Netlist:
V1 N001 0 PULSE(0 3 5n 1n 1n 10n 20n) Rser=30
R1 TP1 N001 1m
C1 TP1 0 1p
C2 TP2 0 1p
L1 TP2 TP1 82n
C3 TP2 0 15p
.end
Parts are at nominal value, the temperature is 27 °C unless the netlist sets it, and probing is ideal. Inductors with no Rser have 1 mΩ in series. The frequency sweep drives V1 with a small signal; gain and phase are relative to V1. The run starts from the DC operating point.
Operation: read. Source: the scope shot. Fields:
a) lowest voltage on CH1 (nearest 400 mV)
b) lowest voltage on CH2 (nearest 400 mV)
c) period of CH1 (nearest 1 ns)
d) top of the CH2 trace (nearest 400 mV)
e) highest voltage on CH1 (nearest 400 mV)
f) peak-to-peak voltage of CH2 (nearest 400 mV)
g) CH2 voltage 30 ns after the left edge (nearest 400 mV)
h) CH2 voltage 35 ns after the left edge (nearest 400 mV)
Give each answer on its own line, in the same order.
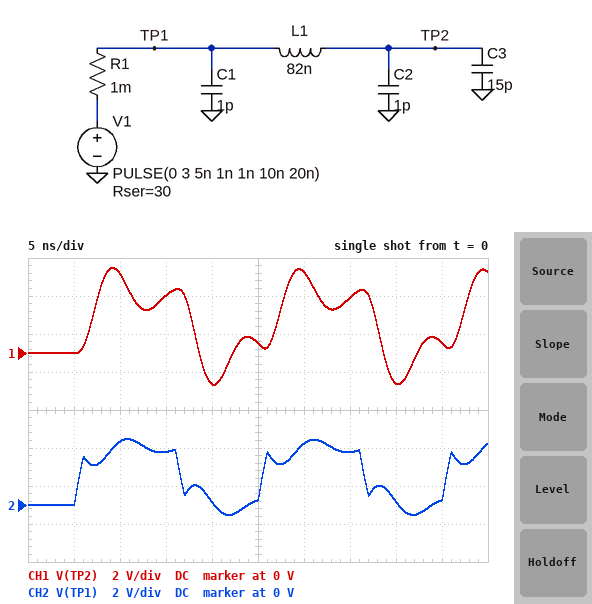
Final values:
-1.6 V
-400 mV
20 ns
3.6 V
4.4 V
4.0 V
3.2 V
2.8 V
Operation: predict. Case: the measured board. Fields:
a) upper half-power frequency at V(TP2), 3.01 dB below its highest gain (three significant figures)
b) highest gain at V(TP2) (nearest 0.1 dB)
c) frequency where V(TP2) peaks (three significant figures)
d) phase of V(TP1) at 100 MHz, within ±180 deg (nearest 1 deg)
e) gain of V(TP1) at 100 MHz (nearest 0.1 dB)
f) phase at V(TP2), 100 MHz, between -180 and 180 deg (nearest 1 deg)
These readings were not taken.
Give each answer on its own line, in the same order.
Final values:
161 MHz
7.7 dB
133 MHz
-33 deg
-1.5 dB
-33 deg
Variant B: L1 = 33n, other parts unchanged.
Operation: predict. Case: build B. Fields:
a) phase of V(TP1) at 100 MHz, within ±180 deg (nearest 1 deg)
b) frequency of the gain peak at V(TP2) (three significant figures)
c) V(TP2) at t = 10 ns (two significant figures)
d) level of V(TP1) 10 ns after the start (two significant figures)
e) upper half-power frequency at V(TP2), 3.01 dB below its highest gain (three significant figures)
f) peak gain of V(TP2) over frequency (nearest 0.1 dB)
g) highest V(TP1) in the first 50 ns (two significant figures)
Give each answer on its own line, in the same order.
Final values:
-22 deg
196 MHz
2.7 V
3.1 V
263 MHz
4.0 dB
3.4 V
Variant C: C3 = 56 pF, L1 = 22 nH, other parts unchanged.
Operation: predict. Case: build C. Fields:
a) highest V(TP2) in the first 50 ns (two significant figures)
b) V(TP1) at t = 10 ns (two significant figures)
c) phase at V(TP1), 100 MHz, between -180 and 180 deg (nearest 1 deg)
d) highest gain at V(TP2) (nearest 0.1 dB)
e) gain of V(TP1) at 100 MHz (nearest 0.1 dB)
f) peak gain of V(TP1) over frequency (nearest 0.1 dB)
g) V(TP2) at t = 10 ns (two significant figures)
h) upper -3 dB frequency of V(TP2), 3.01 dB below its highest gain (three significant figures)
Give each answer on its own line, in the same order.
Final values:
3.1 V
2.8 V
-65 deg
0 dB
-7.5 dB
0 dB
3.0 V
130 MHz
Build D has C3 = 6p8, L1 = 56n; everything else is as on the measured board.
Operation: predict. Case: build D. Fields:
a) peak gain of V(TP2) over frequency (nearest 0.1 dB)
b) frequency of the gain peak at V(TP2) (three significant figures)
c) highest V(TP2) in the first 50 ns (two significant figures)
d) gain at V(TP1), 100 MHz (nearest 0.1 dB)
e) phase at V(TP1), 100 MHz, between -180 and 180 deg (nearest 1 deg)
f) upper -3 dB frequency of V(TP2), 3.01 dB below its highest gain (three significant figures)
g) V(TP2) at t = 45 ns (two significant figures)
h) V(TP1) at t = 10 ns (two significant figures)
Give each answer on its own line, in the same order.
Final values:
9.1 dB
235 MHz
4.5 V
-0.2 dB
-11 deg
275 MHz
290 mV
2.9 V
